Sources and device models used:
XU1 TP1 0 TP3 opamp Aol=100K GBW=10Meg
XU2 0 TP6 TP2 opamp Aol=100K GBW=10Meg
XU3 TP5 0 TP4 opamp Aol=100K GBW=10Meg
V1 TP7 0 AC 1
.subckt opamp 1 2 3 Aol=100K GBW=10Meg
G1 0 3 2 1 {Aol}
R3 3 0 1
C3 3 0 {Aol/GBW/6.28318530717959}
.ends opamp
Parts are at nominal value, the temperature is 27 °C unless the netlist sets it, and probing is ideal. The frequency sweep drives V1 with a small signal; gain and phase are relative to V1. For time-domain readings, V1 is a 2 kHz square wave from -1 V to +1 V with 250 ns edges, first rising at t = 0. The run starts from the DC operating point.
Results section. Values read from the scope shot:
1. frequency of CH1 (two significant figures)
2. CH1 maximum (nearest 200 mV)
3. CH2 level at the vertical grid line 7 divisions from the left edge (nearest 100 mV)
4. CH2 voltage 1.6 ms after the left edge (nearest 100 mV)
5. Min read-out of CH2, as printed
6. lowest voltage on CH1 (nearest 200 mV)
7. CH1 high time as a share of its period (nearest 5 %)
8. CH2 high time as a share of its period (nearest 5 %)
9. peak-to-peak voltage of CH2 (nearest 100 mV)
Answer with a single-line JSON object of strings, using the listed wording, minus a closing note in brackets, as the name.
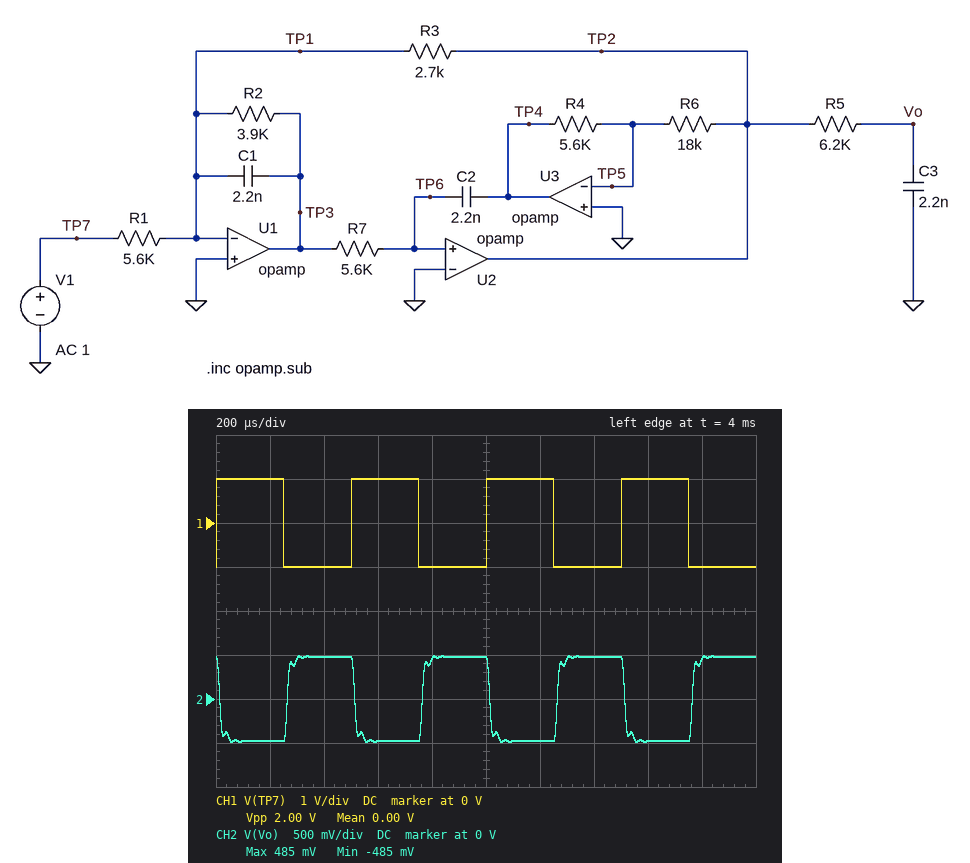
{"frequency of CH1": "2.0 kHz", "CH1 maximum": "1.0 V", "CH2 level at the vertical grid line 7 divisions from the left edge": "500 mV", "CH2 voltage 1.6 ms after the left edge": "-500 mV", "Min read-out of CH2, as printed": "-485 mV", "lowest voltage on CH1": "-1.0 V", "CH1 high time as a share of its period": "50 %", "CH2 high time as a share of its period": "50 %", "peak-to-peak voltage of CH2": "1.0 V"}
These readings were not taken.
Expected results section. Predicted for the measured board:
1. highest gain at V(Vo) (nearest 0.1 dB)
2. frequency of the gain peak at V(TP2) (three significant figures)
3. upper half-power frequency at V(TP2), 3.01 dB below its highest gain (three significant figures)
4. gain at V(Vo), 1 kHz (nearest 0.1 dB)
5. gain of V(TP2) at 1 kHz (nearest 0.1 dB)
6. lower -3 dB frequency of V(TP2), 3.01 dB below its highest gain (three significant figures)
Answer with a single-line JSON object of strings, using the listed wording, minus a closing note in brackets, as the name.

{"highest gain at V(Vo)": "-6.3 dB", "frequency of the gain peak at V(TP2)": "30.6 kHz", "upper half-power frequency at V(TP2), 3.01 dB below its highest gain": "39.0 kHz", "gain at V(Vo), 1 kHz": "-6.4 dB", "gain of V(TP2) at 1 kHz": "-6.3 dB", "lower -3 dB frequency of V(TP2), 3.01 dB below its highest gain": "18.9 kHz"}
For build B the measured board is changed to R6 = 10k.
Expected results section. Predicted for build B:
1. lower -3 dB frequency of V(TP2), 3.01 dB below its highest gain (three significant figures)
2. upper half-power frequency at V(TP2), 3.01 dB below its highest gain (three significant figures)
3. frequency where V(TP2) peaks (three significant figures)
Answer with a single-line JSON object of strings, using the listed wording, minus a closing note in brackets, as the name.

{"lower -3 dB frequency of V(TP2), 3.01 dB below its highest gain": "4.63 kHz", "upper half-power frequency at V(TP2), 3.01 dB below its highest gain": "29.5 kHz", "frequency where V(TP2) peaks": "21.1 kHz"}
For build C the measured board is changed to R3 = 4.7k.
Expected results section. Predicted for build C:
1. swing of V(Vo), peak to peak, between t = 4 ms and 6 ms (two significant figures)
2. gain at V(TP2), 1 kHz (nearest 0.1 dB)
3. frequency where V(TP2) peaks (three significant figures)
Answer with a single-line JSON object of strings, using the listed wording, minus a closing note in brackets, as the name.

{"swing of V(Vo), peak to peak, between t = 4 ms and 6 ms": "1.7 V", "gain at V(TP2), 1 kHz": "-1.5 dB", "frequency where V(TP2) peaks": "21.6 kHz"}
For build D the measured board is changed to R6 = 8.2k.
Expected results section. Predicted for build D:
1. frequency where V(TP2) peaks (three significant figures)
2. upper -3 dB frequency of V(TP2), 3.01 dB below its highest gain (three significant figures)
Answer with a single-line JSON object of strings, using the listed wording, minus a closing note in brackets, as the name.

{"frequency where V(TP2) peaks": "18.3 kHz", "upper -3 dB frequency of V(TP2), 3.01 dB below its highest gain": "26.7 kHz"}
